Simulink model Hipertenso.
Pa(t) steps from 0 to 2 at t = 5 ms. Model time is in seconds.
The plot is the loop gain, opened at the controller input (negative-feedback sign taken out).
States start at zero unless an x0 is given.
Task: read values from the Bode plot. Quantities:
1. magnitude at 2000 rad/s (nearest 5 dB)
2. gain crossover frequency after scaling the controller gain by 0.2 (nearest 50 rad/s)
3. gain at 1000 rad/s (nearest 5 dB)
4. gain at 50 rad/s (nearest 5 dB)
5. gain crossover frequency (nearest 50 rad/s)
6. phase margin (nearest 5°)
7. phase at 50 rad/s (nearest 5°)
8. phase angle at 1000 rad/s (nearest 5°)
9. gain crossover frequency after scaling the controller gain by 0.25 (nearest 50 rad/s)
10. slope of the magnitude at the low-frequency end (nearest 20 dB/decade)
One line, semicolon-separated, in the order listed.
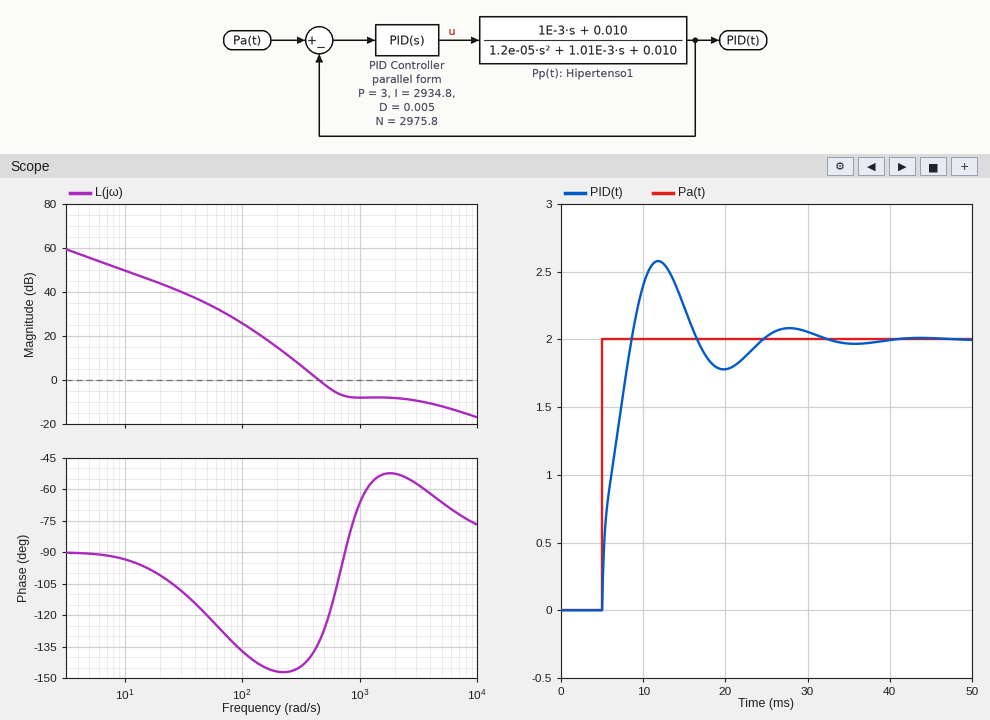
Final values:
-10 dB; 200 rad/s; -10 dB; 35 dB; 450 rad/s; 45°; -120°; -65°; 250 rad/s; -20 dB/decade
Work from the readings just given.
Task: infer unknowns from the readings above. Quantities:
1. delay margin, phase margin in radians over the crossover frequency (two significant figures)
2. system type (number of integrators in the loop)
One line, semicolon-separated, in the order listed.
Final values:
0.0017 s; 1
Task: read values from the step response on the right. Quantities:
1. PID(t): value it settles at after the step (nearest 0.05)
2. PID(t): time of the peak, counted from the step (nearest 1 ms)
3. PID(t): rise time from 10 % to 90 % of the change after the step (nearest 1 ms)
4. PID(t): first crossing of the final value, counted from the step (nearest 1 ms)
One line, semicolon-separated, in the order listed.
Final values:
2.00; 7 ms; 3 ms; 4 ms
